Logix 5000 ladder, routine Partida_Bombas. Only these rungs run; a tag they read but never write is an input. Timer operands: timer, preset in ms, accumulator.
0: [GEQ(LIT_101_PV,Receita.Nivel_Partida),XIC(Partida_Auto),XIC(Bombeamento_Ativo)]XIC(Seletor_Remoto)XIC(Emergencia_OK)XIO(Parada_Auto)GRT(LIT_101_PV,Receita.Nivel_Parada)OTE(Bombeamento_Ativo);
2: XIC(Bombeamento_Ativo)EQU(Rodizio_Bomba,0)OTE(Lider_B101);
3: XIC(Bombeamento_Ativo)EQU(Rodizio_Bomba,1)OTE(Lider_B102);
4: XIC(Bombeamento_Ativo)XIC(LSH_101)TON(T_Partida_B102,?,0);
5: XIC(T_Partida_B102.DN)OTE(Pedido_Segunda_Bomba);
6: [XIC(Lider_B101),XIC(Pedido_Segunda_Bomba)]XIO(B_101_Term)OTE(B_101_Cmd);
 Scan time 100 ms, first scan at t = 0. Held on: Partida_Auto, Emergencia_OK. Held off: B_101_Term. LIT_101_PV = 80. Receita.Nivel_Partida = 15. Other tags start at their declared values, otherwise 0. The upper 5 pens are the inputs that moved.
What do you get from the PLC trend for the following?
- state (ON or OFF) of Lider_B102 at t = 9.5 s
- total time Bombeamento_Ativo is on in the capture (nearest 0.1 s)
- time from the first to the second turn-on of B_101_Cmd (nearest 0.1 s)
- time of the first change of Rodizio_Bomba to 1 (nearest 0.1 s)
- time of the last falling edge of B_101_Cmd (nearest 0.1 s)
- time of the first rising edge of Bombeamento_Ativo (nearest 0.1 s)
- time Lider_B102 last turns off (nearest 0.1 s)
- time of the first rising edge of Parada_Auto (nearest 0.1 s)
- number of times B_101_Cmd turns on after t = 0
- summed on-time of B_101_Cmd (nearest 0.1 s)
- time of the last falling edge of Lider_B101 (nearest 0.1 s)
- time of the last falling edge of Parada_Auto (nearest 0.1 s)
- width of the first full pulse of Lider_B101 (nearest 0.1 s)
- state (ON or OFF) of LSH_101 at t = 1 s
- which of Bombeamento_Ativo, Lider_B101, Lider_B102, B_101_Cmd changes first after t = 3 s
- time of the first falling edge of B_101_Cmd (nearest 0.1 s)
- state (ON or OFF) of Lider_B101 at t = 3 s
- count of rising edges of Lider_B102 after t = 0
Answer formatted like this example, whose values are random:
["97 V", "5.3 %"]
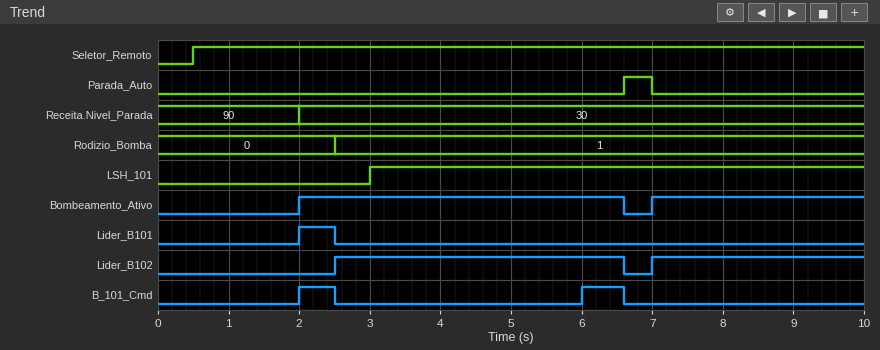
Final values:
["ON", "7.6 s", "4.0 s", "2.5 s", "6.6 s", "2.0 s", "6.6 s", "6.6 s", "2", "1.1 s", "2.5 s", "7.0 s", "0.5 s", "OFF", "B_101_Cmd", "2.5 s", "OFF", "2"]
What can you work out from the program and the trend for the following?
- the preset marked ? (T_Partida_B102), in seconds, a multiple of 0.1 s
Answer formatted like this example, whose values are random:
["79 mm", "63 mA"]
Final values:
["3.0 s"]
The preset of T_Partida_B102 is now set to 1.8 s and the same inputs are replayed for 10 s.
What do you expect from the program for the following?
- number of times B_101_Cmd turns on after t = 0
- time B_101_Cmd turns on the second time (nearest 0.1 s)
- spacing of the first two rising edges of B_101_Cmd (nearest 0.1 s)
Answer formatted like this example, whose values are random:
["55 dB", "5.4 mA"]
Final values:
["3", "4.8 s", "2.8 s"]
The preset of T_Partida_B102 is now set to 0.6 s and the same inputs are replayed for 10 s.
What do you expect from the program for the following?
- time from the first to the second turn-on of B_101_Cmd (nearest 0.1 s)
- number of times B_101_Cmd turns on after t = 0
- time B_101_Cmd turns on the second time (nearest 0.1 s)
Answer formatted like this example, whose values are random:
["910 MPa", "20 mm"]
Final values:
["1.6 s", "3", "3.6 s"]
